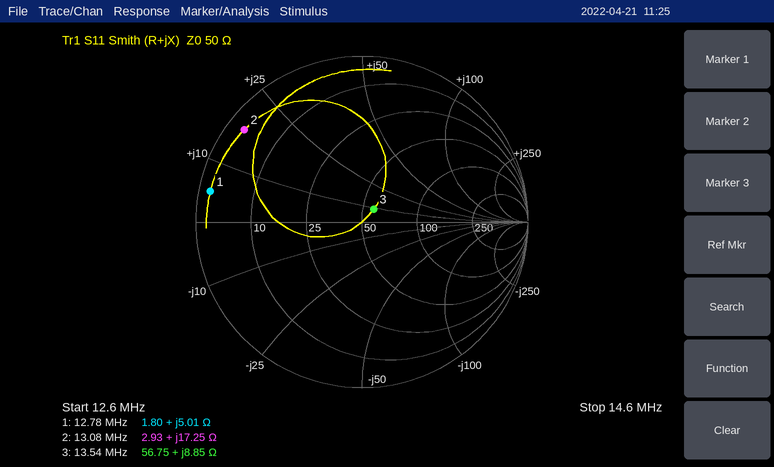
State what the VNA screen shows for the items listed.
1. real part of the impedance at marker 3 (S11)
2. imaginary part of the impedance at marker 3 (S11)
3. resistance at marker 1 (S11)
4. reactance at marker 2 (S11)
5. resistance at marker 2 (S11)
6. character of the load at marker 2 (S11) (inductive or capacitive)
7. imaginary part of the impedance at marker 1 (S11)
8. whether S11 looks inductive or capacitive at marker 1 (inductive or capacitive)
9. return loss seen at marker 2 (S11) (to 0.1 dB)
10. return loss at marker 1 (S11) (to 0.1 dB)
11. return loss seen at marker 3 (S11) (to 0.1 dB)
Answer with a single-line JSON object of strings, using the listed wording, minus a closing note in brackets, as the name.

{"real part of the impedance at marker 3": "56.75 Ω", "imaginary part of the impedance at marker 3": "+8.85 Ω", "resistance at marker 1": "1.80 Ω", "reactance at marker 2": "+17.25 Ω", "resistance at marker 2": "2.93 Ω", "character of the load at marker 2 (S11)": "inductive", "imaginary part of the impedance at marker 1": "+5.01 Ω", "whether S11 looks inductive or capacitive at marker 1": "inductive", "return loss seen at marker 2 (S11)": "0.9 dB", "return loss at marker 1 (S11)": "0.6 dB", "return loss seen at marker 3 (S11)": "19.7 dB"}
